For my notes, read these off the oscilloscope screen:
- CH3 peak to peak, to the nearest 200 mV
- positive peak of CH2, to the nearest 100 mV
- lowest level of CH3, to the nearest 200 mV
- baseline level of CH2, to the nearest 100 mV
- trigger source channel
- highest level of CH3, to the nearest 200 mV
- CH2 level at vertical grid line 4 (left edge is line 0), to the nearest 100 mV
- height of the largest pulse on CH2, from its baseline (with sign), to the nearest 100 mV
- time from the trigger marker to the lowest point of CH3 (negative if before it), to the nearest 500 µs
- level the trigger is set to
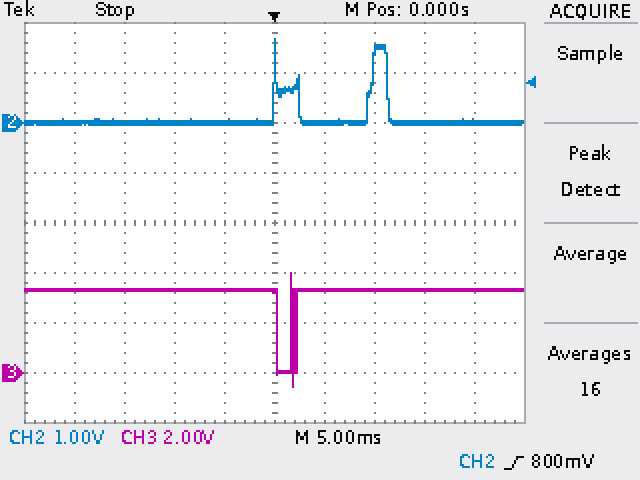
4.6 V
1.7 V
-600 mV
0.0 V
CH2
4.0 V
0.0 V
+1.7 V
+2.0 ms
800 mV
